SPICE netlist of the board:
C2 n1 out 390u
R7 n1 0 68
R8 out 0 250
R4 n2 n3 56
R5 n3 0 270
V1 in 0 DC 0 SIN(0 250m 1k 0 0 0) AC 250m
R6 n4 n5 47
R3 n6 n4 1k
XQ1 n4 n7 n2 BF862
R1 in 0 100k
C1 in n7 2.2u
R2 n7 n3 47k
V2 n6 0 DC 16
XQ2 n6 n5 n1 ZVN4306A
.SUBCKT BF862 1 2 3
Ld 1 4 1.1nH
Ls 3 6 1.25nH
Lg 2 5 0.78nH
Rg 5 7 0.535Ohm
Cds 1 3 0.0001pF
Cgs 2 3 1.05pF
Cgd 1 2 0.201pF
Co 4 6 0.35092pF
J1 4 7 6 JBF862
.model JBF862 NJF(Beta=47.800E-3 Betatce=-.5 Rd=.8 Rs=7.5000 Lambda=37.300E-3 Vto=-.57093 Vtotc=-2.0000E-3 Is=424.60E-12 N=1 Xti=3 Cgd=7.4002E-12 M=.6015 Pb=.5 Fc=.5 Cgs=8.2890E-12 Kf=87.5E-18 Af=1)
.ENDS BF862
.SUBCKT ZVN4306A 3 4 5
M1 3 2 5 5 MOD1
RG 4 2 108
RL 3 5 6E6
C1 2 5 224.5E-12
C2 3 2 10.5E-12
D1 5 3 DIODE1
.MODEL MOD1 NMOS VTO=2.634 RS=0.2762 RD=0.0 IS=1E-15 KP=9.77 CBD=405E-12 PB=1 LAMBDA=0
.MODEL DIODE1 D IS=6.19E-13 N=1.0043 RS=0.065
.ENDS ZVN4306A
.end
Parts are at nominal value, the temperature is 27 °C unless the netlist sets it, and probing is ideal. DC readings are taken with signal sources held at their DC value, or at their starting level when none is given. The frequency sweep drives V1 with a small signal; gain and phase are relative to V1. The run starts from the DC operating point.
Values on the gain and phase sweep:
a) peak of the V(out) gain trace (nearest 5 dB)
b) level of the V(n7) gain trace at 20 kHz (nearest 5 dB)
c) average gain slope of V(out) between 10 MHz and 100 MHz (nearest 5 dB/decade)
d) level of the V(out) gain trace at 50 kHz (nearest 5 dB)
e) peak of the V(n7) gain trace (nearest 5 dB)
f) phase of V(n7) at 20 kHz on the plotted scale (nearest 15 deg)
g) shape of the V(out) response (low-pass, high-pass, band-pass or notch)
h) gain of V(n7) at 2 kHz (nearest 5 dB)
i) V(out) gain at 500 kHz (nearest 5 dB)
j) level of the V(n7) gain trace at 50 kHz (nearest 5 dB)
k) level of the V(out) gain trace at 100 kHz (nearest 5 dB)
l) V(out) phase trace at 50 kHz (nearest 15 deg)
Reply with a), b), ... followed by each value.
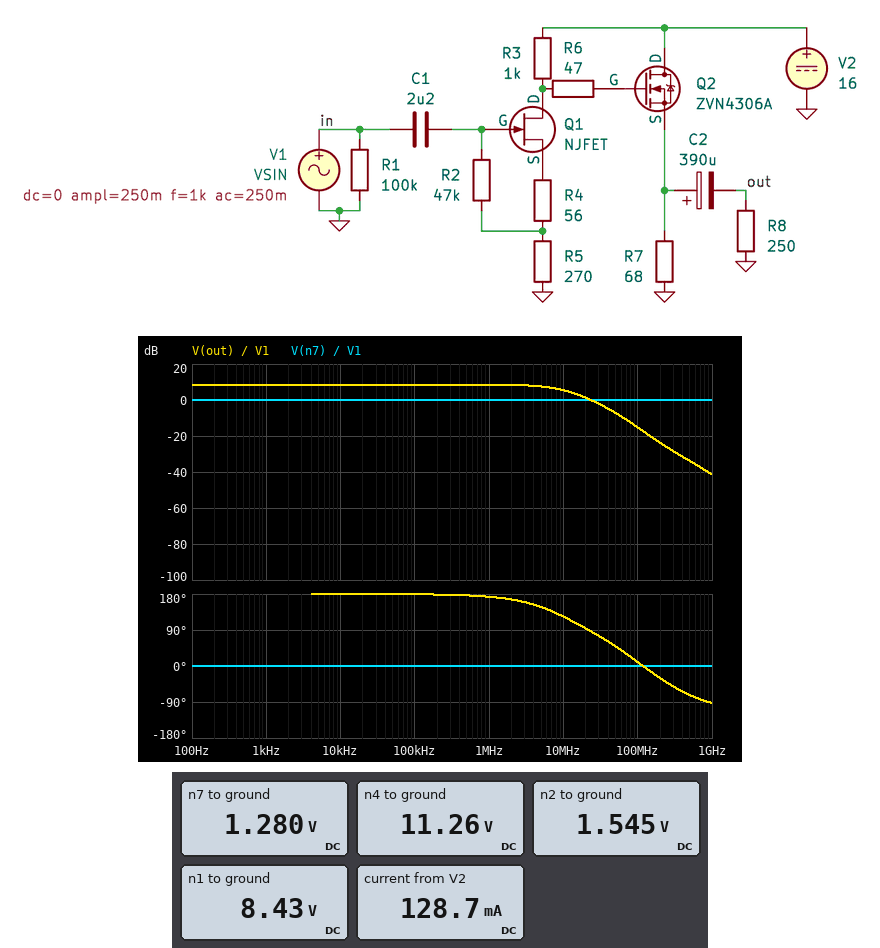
a) 10 dB
b) 0 dB
c) -20 dB/decade
d) 10 dB
e) 0 dB
f) 0 deg
g) low-pass
h) 0 dB
i) 10 dB
j) 0 dB
k) 10 dB
l) 180 deg
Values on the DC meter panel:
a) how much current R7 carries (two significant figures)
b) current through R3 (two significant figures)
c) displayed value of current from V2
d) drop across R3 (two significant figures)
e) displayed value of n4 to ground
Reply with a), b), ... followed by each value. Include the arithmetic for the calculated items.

a) (8.43 V) / 68 Ω = 120 mA
b) (16 V - 11.26 V) / 1 kΩ = 4.7 mA
c) 128.7 mA
d) 16 V - 11.26 V = 4.7 V
e) 11.26 V
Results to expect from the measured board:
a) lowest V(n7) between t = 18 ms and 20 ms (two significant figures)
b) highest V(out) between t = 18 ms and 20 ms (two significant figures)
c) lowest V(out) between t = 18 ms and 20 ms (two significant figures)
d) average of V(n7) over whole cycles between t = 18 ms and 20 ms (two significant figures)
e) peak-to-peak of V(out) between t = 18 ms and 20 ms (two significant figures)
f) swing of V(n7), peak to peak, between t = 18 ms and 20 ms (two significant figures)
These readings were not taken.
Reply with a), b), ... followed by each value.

a) 1.0 V
b) 670 mV
c) -670 mV
d) 1.3 V
e) 1.3 V
f) 500 mV
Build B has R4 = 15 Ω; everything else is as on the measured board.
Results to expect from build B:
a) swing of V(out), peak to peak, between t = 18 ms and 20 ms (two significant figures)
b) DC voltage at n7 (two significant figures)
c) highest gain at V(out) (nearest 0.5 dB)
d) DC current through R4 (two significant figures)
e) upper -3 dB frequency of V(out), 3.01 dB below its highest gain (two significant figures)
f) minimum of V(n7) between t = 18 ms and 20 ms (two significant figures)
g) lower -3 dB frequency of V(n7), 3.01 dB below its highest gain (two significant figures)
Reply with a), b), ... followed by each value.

a) 1.5 V
b) 2.3 V
c) 9.5 dB
d) 8.4 mA
e) 9.0 MHz
f) 2.0 V
g) 250 mHz
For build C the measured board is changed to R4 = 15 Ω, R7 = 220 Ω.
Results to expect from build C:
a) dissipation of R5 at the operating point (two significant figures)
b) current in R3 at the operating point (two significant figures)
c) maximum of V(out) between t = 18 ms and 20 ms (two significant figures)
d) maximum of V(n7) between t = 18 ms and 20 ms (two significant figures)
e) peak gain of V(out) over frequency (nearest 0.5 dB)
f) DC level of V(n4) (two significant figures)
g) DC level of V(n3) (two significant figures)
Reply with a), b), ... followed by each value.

a) 19 mW
b) 8.4 mA
c) 760 mV
d) 2.5 V
e) 9.5 dB
f) 7.6 V
g) 2.3 V
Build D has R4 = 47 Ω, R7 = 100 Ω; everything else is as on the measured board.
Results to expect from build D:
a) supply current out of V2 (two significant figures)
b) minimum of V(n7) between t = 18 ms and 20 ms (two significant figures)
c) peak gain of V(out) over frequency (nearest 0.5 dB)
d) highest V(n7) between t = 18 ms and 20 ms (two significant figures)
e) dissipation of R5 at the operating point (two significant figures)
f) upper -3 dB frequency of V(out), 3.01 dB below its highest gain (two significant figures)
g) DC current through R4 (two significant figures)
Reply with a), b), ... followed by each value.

a) 85 mA
b) 1.2 V
c) 9.0 dB
d) 1.7 V
e) 7.4 mW
f) 10 MHz
g) 5.2 mA
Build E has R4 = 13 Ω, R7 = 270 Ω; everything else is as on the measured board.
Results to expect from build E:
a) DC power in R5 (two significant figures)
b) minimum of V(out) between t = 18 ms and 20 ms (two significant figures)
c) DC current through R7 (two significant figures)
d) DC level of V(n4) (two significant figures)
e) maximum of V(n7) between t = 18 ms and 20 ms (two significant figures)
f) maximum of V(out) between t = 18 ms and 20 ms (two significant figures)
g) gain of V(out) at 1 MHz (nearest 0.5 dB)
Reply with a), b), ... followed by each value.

a) 20 mW
b) -760 mV
c) 17 mA
d) 7.3 V
e) 2.6 V
f) 770 mV
g) 9.5 dB
